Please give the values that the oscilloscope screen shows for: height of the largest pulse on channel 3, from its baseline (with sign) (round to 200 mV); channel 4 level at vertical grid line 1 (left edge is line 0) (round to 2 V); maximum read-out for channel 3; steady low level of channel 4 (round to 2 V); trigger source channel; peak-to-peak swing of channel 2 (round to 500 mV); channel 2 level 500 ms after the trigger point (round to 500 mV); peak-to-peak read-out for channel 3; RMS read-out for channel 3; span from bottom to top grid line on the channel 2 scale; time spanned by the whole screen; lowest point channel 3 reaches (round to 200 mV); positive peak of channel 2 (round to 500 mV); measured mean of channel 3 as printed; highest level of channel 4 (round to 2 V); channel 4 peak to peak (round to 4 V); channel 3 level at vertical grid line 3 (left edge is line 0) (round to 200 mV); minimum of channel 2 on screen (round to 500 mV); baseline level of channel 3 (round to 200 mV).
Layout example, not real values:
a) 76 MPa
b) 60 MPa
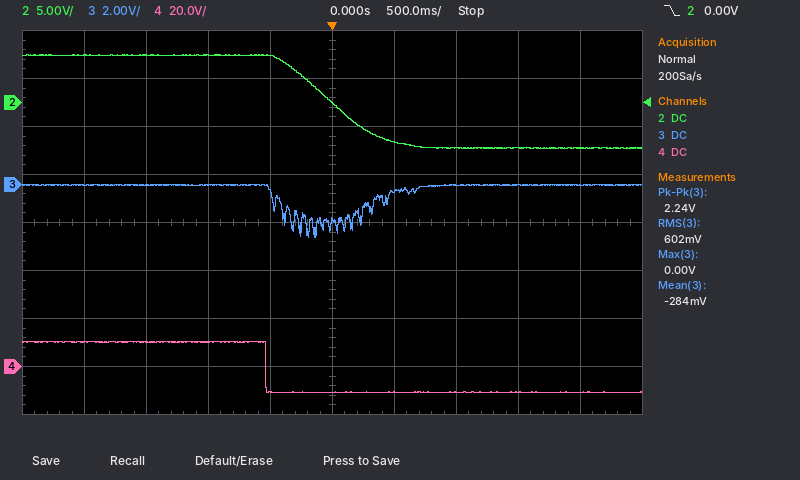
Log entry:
a) -2.2 V
b) 10 V
c) 0.00 V
d) -10 V
e) channel 2
f) 10.0 V
g) -4.0 V
h) 2.24 V
i) 602 mV
j) 40 V
k) 5 s
l) -2.2 V
m) 5.0 V
n) -284 mV
o) 10 V
p) 20 V
q) 0.0 V
r) -5.0 V
s) 0.0 V
